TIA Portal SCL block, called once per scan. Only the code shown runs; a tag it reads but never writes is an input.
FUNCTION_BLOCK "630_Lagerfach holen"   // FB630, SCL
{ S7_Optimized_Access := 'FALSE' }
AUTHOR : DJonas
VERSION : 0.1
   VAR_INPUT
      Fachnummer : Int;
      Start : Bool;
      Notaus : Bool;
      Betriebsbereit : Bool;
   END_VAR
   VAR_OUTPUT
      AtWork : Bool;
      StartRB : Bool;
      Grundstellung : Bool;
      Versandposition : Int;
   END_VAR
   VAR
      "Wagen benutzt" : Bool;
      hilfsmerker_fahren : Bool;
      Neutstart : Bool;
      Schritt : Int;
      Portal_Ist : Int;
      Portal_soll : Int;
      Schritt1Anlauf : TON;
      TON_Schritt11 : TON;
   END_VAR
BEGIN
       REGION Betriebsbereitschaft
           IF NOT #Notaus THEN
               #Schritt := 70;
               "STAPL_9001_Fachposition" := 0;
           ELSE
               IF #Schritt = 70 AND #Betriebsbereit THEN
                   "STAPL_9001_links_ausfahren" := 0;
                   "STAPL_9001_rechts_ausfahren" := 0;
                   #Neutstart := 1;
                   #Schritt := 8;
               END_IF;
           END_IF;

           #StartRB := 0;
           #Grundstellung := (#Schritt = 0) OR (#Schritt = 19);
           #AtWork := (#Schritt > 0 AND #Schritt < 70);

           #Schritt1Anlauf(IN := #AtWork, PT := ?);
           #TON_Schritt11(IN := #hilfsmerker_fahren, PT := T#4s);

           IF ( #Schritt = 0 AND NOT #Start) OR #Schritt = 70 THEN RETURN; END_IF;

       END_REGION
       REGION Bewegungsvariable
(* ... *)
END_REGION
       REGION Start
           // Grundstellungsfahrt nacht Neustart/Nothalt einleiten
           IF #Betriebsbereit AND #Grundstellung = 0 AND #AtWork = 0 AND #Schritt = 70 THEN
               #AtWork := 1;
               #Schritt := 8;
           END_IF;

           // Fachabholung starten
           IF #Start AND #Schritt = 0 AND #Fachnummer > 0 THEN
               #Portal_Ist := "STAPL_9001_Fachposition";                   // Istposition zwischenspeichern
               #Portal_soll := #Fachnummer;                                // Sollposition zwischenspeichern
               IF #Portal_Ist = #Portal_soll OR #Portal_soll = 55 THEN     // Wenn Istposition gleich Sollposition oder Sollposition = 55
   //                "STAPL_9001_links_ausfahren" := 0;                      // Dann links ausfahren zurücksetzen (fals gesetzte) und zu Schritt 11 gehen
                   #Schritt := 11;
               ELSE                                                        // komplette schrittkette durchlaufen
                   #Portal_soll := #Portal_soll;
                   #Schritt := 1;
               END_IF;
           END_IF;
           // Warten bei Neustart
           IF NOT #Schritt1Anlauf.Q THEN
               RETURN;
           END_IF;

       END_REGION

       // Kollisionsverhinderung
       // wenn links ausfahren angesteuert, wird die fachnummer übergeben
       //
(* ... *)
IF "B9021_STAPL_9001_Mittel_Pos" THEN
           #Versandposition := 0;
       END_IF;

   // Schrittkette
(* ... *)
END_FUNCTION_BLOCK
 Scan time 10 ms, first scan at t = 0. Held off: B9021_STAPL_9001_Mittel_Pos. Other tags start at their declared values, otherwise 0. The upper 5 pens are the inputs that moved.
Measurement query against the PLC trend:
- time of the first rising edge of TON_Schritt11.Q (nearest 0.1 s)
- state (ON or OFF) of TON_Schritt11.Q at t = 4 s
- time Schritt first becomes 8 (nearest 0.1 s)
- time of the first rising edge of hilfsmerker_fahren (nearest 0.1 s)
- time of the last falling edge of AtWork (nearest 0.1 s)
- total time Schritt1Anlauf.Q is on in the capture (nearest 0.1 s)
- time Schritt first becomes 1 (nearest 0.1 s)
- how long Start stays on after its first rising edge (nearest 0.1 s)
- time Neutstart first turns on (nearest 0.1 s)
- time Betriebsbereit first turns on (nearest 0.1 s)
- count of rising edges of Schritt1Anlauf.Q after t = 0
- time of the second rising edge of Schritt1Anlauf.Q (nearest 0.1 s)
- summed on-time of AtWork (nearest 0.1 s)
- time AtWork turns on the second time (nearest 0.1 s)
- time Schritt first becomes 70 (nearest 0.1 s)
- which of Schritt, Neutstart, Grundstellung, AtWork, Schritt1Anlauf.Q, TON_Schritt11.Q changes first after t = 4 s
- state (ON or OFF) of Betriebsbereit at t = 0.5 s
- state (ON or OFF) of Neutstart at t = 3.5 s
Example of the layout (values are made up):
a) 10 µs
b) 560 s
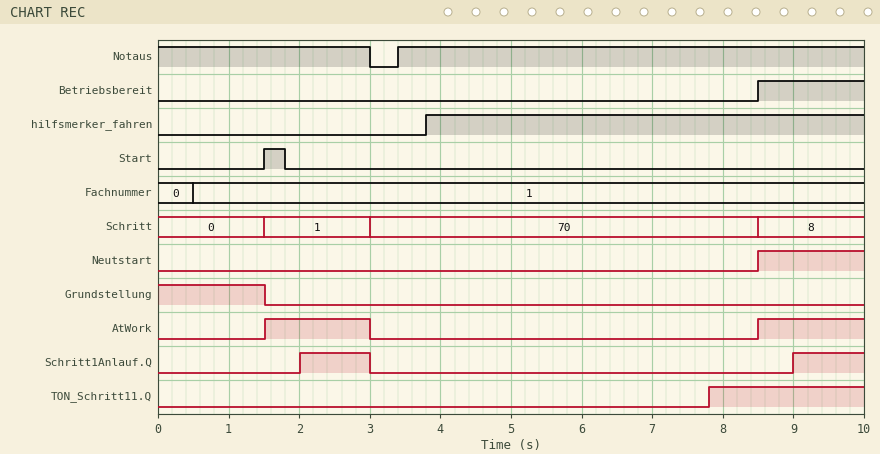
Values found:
a) 7.8 s
b) OFF
c) 8.5 s
d) 3.8 s
e) 3.0 s
f) 2.0 s
g) 1.5 s
h) 0.3 s
i) 8.5 s
j) 8.5 s
k) 2
l) 9.0 s
m) 3.0 s
n) 8.5 s
o) 3.0 s
p) TON_Schritt11.Q
q) OFF
r) OFF
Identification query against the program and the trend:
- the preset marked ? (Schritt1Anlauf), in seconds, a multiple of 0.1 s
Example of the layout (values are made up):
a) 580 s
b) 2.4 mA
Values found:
a) 0.5 s
